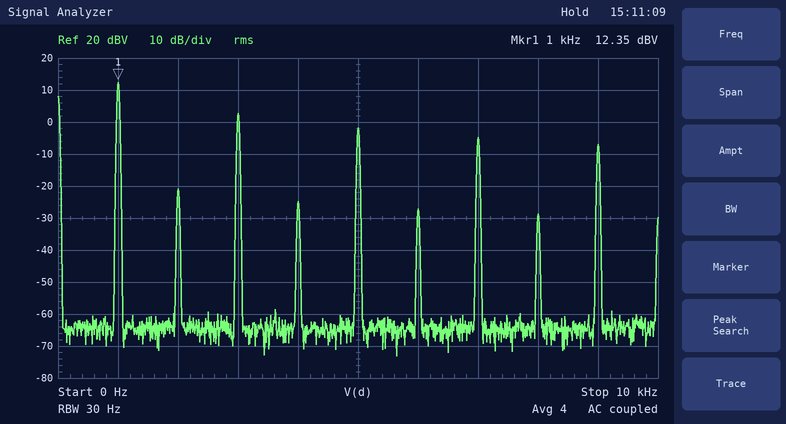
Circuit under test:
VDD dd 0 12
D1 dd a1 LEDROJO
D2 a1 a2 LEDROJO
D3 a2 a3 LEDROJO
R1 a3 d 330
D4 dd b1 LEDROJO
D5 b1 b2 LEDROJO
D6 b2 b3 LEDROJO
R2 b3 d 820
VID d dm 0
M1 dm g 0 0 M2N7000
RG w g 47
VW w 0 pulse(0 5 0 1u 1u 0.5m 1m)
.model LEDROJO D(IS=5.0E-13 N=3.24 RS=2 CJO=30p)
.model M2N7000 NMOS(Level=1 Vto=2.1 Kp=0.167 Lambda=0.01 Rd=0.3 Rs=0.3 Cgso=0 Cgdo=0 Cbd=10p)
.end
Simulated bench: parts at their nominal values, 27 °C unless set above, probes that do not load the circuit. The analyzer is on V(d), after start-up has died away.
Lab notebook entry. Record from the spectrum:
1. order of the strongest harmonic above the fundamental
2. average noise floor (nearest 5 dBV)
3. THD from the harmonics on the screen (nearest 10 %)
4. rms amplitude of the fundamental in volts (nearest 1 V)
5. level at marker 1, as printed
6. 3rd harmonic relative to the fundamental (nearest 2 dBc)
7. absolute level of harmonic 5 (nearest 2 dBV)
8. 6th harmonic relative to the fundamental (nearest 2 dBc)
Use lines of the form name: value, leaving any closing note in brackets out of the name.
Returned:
order of the strongest harmonic above the fundamental: 3
average noise floor: -65 dBV
THD from the harmonics on the screen: 40 %
rms amplitude of the fundamental in volts: 4 V
level at marker 1, as printed: 12.35 dBV
3rd harmonic relative to the fundamental: -10 dBc
absolute level of harmonic 5: -2 dBV
6th harmonic relative to the fundamental: -40 dBc
